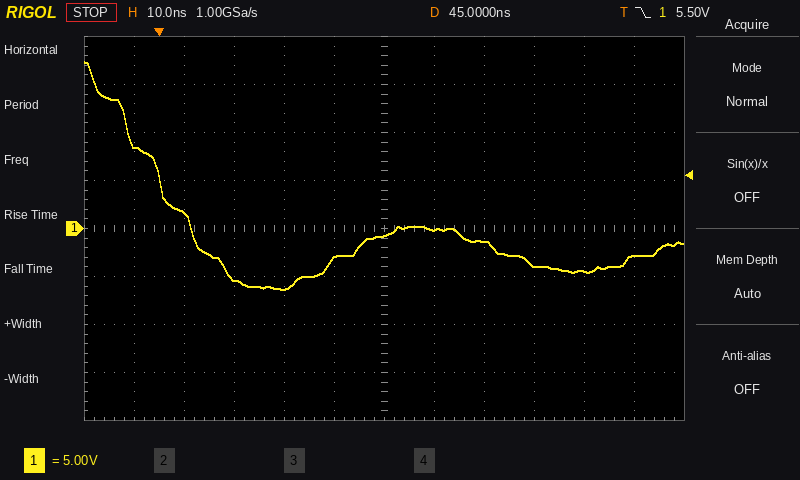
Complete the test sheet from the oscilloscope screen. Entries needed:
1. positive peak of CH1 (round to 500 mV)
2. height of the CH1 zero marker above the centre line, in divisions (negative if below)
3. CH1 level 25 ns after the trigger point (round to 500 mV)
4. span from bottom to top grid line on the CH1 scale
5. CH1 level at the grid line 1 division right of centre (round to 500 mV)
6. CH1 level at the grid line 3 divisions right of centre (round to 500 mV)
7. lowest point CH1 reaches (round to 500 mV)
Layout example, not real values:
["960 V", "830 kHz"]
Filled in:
["17.5 V", "0.0 div", "-6.5 V", "40 V", "0.0 V", "-4.0 V", "-6.5 V"]
